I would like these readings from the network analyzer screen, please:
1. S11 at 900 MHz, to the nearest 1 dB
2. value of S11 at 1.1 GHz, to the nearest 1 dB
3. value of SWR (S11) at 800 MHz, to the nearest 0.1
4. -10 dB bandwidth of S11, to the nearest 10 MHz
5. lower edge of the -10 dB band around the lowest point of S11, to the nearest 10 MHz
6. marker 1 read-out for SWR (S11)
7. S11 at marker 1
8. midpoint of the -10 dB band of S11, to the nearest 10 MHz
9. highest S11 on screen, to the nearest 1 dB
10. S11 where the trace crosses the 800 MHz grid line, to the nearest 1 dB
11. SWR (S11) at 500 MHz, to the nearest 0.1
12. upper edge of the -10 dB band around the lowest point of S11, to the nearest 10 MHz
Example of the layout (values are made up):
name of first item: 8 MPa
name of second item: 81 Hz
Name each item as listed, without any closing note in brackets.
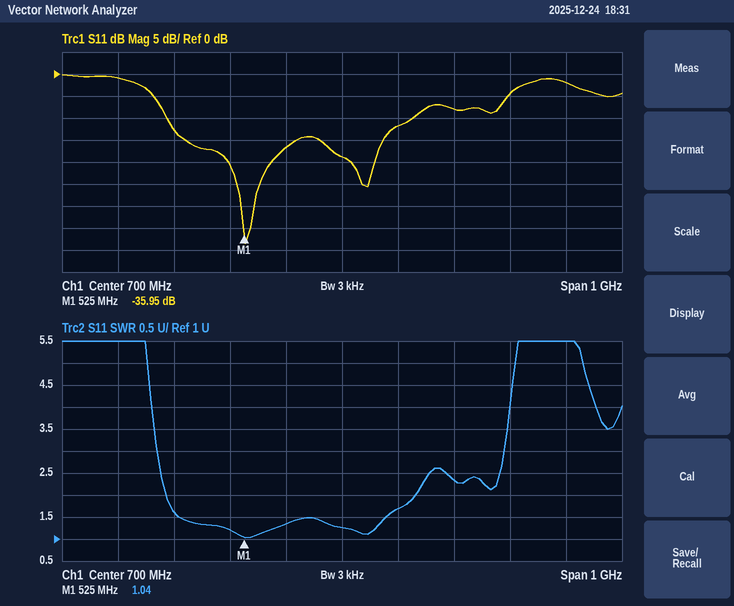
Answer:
S11 at 900 MHz, to the nearest 1 dB: -8 dB
value of S11 at 1.1 GHz, to the nearest 1 dB: -2 dB
value of SWR (S11) at 800 MHz, to the nearest 0.1: 1.7
-10 dB bandwidth of S11, to the nearest 10 MHz: 440 MHz
lower edge of the -10 dB band around the lowest point of S11, to the nearest 10 MHz: 390 MHz
marker 1 read-out for SWR: 1.04
S11 at marker 1: -35.95 dB
midpoint of the -10 dB band of S11, to the nearest 10 MHz: 610 MHz
highest S11 on screen, to the nearest 1 dB: 0 dB
S11 where the trace crosses the 800 MHz grid line, to the nearest 1 dB: -12 dB
SWR (S11) at 500 MHz, to the nearest 0.1: 1.2
upper edge of the -10 dB band around the lowest point of S11, to the nearest 10 MHz: 830 MHz
